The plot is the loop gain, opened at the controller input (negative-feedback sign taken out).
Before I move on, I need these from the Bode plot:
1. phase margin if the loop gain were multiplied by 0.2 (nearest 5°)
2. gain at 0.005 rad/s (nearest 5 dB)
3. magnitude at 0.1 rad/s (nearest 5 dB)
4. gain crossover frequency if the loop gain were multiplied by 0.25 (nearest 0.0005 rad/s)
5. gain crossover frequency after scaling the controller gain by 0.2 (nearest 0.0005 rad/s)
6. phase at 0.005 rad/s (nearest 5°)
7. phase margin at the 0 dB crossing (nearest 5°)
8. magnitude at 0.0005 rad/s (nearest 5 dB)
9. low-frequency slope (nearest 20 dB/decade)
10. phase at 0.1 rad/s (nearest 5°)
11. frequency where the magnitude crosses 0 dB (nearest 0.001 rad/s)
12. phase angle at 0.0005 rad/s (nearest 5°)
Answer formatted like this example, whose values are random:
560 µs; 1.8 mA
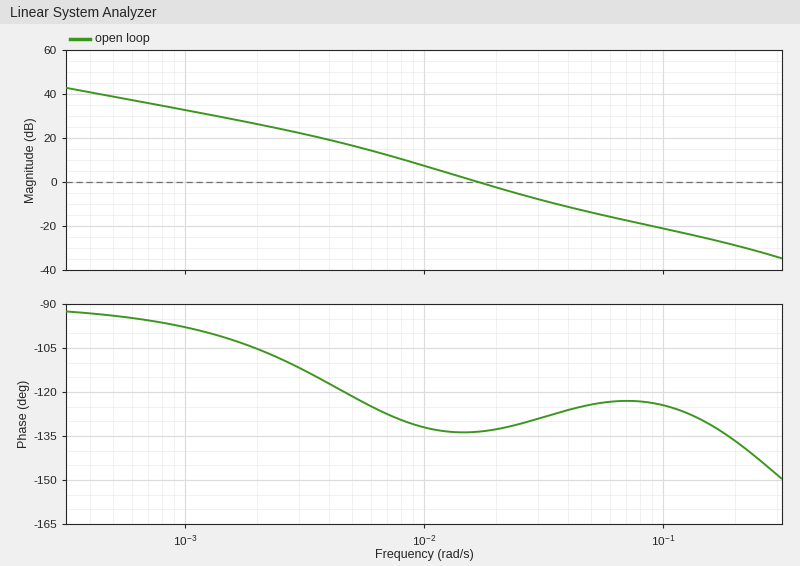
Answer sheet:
55°; 15 dB; -20 dB; 0.0070 rad/s; 0.0060 rad/s; -120°; 45°; 40 dB; -20 dB/decade; -125°; 0.017 rad/s; -95°
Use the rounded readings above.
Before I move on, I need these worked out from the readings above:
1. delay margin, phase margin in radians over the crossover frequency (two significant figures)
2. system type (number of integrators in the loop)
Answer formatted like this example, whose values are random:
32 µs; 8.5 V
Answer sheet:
46 s; 1
